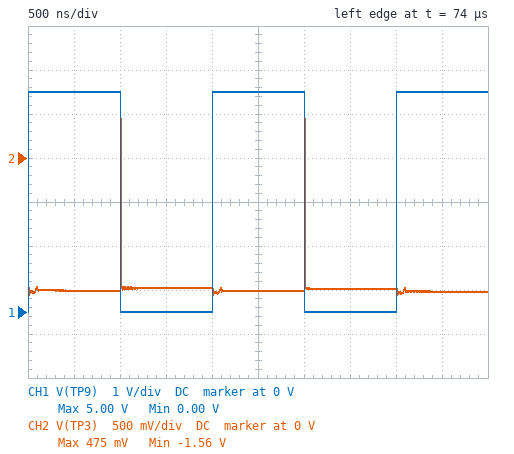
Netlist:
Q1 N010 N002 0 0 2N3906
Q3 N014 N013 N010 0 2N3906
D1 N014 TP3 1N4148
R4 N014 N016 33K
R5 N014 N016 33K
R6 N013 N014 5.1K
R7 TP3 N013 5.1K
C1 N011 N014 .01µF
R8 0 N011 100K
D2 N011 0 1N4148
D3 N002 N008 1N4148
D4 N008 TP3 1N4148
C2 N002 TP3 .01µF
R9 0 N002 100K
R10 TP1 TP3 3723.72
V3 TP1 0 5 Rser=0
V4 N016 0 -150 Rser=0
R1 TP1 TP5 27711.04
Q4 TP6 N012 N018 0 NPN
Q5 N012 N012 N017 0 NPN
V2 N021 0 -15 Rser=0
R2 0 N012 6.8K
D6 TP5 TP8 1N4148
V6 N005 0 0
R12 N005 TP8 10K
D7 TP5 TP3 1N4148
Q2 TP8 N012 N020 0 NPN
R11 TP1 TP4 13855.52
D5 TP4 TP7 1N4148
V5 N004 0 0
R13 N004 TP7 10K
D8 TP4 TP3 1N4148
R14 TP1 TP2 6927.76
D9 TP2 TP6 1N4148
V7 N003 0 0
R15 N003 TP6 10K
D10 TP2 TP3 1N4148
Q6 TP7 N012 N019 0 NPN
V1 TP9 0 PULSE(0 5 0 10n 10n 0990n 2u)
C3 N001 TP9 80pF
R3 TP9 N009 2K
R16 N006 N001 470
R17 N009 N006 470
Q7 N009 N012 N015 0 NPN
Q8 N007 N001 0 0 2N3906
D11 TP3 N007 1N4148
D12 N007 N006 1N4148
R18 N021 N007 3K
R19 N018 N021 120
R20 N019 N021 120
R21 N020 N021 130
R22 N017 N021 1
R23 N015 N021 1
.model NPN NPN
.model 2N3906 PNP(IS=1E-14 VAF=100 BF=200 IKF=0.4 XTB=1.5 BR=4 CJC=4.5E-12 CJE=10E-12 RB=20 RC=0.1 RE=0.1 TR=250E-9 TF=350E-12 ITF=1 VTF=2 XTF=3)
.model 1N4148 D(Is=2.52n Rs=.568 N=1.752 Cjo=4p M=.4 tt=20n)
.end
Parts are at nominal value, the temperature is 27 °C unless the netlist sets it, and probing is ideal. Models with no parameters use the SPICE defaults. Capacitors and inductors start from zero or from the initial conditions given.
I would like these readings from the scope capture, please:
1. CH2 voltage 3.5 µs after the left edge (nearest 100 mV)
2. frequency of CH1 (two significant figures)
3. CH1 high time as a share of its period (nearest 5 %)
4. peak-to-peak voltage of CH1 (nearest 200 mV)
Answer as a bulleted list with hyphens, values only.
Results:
- -1.5 V
- 500 kHz
- 50 %
- 5.0 V
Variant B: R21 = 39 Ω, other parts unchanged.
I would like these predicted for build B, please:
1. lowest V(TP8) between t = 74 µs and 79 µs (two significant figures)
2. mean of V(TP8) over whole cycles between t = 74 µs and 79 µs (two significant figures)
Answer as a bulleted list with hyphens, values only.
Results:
- -4.8 V
- -4.2 V
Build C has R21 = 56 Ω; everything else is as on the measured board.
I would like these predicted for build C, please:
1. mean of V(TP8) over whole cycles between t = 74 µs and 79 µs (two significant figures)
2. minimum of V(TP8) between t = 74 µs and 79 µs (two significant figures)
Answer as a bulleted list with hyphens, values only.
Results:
- -3.2 V
- -3.8 V
